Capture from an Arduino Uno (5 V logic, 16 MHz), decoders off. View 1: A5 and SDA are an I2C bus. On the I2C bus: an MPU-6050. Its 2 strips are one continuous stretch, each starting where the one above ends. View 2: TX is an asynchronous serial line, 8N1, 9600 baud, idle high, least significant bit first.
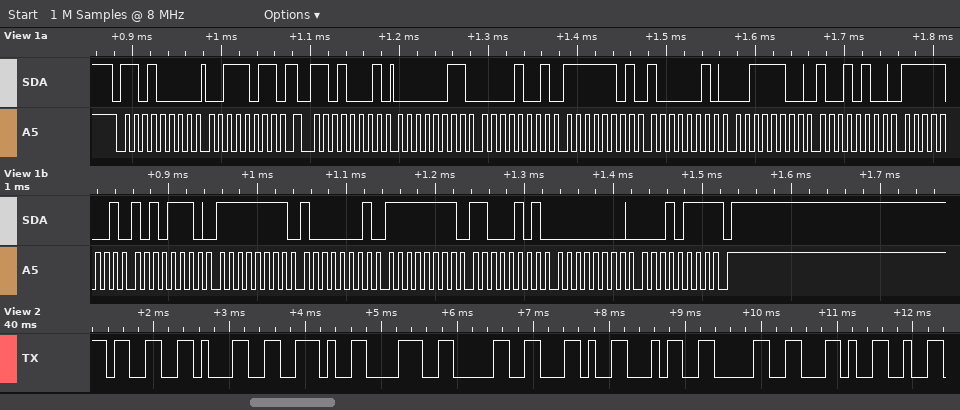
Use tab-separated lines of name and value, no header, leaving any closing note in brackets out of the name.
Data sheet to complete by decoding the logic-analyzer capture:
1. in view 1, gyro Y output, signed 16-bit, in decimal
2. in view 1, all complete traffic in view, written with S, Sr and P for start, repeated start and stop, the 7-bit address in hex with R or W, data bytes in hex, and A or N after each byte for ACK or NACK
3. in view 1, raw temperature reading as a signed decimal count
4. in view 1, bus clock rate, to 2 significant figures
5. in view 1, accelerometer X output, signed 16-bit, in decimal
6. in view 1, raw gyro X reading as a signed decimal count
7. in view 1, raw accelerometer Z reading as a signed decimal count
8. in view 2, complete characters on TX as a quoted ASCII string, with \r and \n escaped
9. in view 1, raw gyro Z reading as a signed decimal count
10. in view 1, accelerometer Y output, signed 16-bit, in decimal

in view 1, gyro Y output, signed 16-bit, in decimal	-59
in view 1, all complete traffic in view, written with S, Sr and P for start, repeated start and stop, the 7-bit address in hex with R or W, data bytes in hex, and A or N after each byte for ACK or NACK	S 68W A 3B A Sr 68R A 03 A 09 A FD A 82 A 3C A 94 A F9 A AE A FF A 81 A FF A C5 A 00 A 17 N P
in view 1, raw temperature reading as a signed decimal count	-1618
in view 1, bus clock rate, to 2 significant figures	100 kHz
in view 1, accelerometer X output, signed 16-bit, in decimal	777
in view 1, raw gyro X reading as a signed decimal count	-127
in view 1, raw accelerometer Z reading as a signed decimal count	15508
in view 2, complete characters on TX as a quoted ASCII string, with \r and \n escaped	"31.80,40,"
in view 1, raw gyro Z reading as a signed decimal count	23
in view 1, accelerometer Y output, signed 16-bit, in decimal	-638
